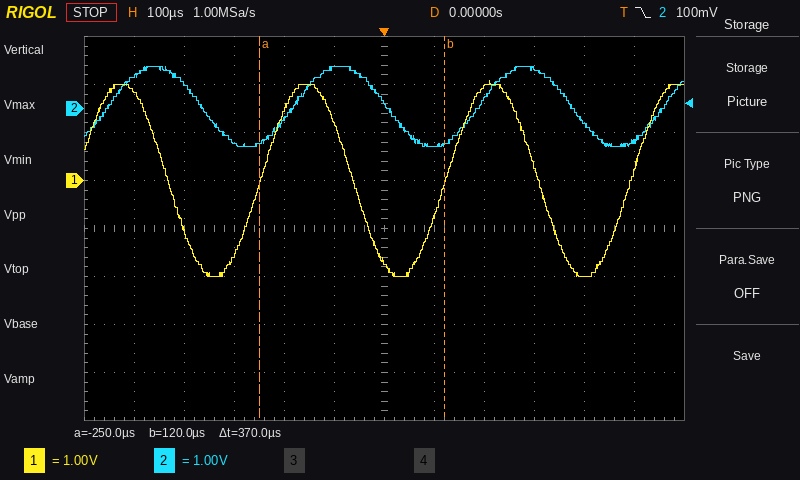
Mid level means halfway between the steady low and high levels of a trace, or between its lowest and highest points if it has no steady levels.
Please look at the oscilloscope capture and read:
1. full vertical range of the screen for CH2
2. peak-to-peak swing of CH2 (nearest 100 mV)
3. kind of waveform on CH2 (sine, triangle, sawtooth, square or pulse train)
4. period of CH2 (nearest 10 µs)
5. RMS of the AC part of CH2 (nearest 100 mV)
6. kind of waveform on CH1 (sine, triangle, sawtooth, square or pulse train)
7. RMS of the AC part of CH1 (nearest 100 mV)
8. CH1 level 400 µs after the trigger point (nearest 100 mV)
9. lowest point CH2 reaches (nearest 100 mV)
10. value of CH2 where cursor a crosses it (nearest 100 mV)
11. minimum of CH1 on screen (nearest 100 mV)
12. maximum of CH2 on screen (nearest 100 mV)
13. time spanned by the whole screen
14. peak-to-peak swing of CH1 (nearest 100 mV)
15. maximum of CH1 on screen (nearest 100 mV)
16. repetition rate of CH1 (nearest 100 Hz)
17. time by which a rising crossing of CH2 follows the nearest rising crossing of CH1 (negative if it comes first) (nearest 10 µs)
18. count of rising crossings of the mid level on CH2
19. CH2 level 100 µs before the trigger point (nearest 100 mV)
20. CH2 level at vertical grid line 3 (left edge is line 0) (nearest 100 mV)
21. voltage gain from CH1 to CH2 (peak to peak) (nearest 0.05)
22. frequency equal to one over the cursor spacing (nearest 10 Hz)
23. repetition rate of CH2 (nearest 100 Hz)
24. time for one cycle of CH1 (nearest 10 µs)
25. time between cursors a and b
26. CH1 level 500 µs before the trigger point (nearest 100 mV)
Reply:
8 V
1.7 V
sine
370 µs
600 mV
sine
1.4 V
-2.0 V
-800 mV
-700 mV
-2.0 V
900 mV
1.2 ms
4.1 V
2.1 V
2.7 kHz
+70 µs
4
800 mV
-700 mV
0.40
2.70 kHz
2.7 kHz
370 µs
370 µs
1.8 V
